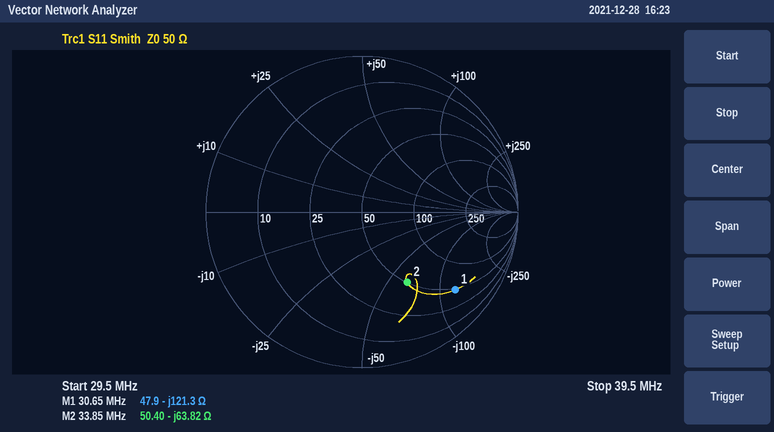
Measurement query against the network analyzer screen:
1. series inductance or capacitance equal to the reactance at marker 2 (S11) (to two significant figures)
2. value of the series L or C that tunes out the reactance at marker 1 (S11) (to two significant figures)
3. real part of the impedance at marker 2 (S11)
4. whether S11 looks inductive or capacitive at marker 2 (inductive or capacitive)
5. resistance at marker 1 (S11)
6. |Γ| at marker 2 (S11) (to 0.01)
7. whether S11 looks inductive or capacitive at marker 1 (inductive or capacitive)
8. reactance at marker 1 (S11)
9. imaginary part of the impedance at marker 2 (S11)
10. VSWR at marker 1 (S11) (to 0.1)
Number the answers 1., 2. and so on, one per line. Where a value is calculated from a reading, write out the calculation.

1. C = 1/(2π × 33.85 MHz × 63.82 Ω) ≈ 74 pF
2. L = 121.3 Ω/(2π × 30.65 MHz) ≈ 630 nH
3. 50.40 Ω
4. capacitive
5. 47.9 Ω
6. 0.54
7. capacitive
8. -121.3 Ω
9. -63.82 Ω
10. 8.0
